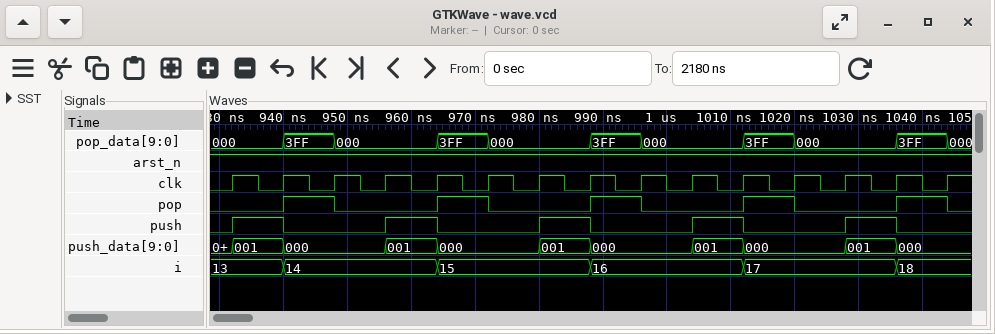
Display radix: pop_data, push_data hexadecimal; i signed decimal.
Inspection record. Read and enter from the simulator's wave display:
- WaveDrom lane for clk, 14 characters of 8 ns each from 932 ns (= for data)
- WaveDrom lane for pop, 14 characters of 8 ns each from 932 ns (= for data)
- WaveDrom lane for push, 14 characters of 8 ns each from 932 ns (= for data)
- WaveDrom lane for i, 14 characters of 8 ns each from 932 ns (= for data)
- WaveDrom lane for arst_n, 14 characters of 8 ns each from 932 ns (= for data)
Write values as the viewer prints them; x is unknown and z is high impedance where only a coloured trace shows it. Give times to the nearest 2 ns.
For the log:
{name: 'clk', wave: 'p.............'}
{name: 'pop', wave: '010.10.10.10.1'}
{name: 'push', wave: '10.10.10.10.10'}
{name: 'i', wave: '==..=..=..=..=', data: '13 14 15 16 17 18'}
{name: 'arst_n', wave: '1.............'}
